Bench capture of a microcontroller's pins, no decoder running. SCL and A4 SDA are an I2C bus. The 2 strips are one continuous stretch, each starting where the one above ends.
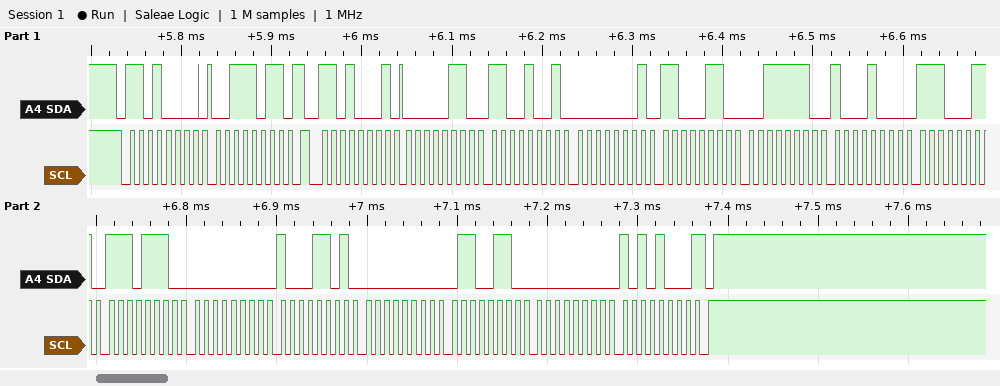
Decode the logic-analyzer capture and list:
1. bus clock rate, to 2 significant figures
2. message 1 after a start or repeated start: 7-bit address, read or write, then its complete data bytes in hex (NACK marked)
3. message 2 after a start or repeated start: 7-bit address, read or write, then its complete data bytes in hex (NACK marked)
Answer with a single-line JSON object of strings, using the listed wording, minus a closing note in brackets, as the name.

{"bus clock rate, to 2 significant figures": "100 kHz", "message 1 after a start or repeated start: 7-bit address, read or write, then its complete data bytes in hex": "0x68 write: 3B", "message 2 after a start or repeated start: 7-bit address, read or write, then its complete data bytes in hex": "0x68 read: 06 C9 01 C6 3E 88 E3 EE 00 8D 00 66 00 A8 NACK"}
